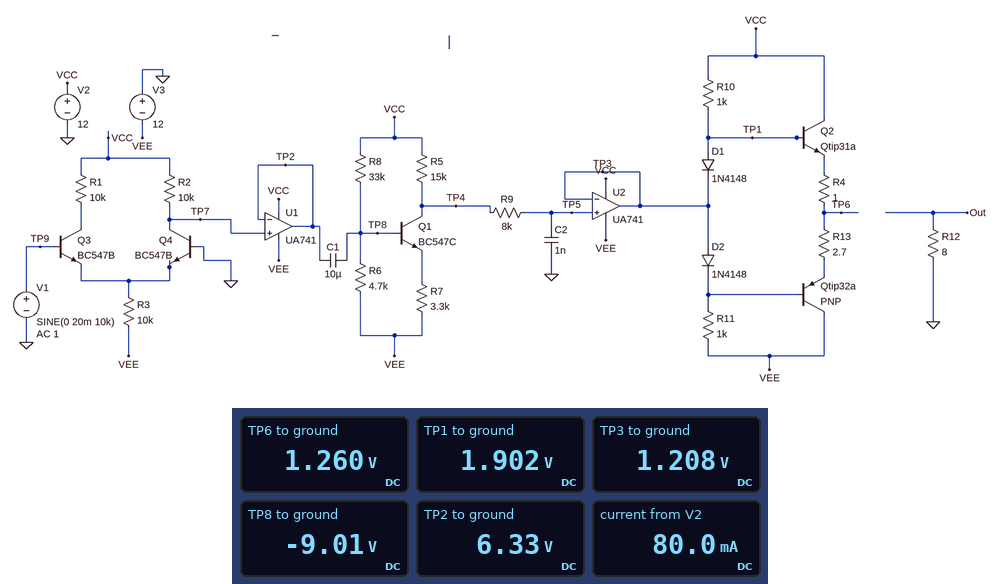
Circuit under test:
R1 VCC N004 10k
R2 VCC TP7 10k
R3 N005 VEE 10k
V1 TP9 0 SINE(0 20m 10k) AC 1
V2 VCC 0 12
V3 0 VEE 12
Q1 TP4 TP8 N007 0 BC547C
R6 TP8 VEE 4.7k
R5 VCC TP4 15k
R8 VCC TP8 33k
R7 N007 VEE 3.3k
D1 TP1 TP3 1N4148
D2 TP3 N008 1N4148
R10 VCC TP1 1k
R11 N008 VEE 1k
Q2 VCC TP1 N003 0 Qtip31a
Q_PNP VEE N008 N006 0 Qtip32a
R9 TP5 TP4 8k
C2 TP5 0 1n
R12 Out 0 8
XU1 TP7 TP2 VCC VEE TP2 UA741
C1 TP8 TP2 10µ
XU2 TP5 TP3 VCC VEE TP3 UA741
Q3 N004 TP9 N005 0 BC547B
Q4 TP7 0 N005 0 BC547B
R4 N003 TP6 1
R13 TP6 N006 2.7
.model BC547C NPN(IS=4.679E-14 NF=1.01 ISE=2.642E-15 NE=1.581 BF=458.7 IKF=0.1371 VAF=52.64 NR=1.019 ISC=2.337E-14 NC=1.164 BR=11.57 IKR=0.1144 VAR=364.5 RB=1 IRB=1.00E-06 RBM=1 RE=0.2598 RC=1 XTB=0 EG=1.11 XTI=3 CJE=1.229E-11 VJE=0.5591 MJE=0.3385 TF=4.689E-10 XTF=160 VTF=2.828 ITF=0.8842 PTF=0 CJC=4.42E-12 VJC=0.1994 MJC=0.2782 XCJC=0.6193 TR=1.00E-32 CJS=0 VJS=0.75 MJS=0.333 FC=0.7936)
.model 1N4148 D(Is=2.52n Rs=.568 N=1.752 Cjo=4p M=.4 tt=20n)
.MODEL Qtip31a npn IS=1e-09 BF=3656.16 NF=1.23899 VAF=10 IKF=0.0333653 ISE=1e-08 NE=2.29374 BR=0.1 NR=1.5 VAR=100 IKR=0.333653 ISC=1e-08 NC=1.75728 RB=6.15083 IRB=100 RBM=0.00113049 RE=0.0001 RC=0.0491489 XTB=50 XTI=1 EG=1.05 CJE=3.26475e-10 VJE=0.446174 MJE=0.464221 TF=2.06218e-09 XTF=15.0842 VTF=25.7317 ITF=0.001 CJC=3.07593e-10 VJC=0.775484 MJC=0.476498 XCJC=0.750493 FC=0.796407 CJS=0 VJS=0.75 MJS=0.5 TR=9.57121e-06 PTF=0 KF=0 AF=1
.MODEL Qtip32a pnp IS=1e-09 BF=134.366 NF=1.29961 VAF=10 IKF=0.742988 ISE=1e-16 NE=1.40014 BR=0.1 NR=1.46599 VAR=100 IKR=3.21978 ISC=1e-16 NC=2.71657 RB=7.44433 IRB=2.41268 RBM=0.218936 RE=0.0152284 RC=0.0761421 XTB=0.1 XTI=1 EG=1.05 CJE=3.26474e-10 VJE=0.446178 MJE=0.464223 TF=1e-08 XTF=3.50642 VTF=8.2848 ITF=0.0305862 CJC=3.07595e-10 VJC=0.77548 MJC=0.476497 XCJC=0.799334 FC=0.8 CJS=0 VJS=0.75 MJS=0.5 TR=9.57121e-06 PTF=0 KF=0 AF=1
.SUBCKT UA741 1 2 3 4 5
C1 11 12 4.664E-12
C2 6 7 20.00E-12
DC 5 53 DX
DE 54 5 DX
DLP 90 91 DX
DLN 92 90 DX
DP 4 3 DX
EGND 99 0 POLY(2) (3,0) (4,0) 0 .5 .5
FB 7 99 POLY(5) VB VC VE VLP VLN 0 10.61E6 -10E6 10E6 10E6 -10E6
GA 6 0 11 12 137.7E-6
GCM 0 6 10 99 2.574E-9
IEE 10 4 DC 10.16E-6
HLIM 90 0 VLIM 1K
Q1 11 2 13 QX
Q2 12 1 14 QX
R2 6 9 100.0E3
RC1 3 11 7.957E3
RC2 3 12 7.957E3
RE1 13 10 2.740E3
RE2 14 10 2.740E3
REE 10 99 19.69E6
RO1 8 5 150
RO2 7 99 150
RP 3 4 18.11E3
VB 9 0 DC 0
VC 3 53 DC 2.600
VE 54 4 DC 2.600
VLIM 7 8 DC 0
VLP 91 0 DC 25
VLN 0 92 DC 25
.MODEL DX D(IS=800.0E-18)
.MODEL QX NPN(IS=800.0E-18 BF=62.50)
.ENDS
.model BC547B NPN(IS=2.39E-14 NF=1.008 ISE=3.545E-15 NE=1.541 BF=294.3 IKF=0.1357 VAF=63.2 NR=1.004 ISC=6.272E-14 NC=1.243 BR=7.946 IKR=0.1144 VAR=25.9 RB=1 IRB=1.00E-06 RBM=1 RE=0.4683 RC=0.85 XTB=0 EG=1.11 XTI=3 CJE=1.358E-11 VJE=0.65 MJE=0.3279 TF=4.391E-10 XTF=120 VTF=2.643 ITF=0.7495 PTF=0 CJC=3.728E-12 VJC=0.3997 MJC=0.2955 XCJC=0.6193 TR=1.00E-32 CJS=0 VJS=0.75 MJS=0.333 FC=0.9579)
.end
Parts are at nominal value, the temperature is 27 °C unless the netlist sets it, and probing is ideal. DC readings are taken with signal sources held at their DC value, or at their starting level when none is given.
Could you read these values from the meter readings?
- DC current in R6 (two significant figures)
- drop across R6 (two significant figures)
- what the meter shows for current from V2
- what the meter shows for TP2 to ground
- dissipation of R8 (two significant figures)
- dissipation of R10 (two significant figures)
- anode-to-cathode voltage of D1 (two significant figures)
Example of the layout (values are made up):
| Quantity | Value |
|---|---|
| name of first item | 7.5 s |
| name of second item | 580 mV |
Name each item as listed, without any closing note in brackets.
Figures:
| Quantity | Value |
|---|---|
| DC current in R6 | 640 µA |
| drop across R6 | 3.0 V |
| what the meter shows for current from V2 | 80.0 mA |
| what the meter shows for TP2 to ground | 6.33 V |
| dissipation of R8 | 13 mW |
| dissipation of R10 | 100 mW |
| anode-to-cathode voltage of D1 | 690 mV |
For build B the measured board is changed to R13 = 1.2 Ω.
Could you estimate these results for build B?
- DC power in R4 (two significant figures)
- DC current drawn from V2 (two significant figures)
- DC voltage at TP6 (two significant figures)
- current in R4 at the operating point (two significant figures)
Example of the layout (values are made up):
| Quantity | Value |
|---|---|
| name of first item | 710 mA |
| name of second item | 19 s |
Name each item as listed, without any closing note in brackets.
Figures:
| Quantity | Value |
|---|---|
| DC power in R4 | 8.8 mW |
| DC current drawn from V2 | 110 mA |
| DC voltage at TP6 | 1.2 V |
| current in R4 at the operating point | 94 mA |
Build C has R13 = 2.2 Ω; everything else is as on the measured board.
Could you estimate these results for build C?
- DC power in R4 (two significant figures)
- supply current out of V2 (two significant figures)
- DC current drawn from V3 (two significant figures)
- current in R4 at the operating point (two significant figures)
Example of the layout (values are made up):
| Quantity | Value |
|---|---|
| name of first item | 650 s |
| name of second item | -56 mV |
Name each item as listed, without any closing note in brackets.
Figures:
| Quantity | Value |
|---|---|
| DC power in R4 | 5.2 mW |
| supply current out of V2 | 87 mA |
| DC current drawn from V3 | 90 mA |
| current in R4 at the operating point | 72 mA |
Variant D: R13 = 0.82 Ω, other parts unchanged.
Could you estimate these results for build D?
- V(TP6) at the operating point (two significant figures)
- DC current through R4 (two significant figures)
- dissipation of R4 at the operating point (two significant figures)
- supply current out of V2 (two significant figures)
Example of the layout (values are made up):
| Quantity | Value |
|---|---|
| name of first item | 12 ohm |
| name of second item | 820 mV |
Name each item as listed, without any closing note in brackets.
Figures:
| Quantity | Value |
|---|---|
| V(TP6) at the operating point | 1.2 V |
| DC current through R4 | 110 mA |
| dissipation of R4 at the operating point | 11 mW |
| supply current out of V2 | 120 mA |
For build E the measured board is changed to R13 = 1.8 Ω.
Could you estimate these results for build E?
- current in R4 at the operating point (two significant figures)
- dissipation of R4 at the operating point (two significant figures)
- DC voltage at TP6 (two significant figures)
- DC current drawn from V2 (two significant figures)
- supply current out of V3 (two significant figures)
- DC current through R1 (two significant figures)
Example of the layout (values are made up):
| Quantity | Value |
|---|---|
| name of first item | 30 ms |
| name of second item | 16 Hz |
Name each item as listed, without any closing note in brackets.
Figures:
| Quantity | Value |
|---|---|
| current in R4 at the operating point | 79 mA |
| dissipation of R4 at the operating point | 6.3 mW |
| DC voltage at TP6 | 1.2 V |
| DC current drawn from V2 | 94 mA |
| supply current out of V3 | 97 mA |
| DC current through R1 | 570 µA |
